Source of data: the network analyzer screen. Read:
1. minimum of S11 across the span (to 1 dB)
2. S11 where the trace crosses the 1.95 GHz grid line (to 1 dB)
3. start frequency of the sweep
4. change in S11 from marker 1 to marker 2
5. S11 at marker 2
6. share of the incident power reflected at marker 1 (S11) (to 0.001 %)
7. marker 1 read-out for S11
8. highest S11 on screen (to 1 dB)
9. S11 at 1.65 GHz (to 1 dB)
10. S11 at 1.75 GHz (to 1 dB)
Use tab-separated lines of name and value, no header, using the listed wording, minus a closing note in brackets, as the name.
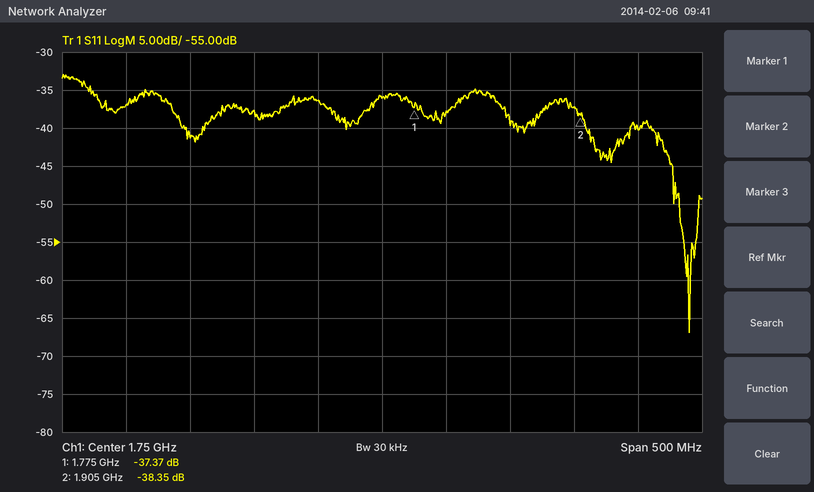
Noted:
minimum of S11 across the span	-67 dB
S11 where the trace crosses the 1.95 GHz grid line	-40 dB
start frequency of the sweep	1.5 GHz
change in S11 from marker 1 to marker 2	-0.98 dB
S11 at marker 2	-38.35 dB
share of the incident power reflected at marker 1 (S11)	0.018 %
marker 1 read-out for S11	-37.37 dB
highest S11 on screen	-33 dB
S11 at 1.65 GHz	-38 dB
S11 at 1.75 GHz	-36 dB
